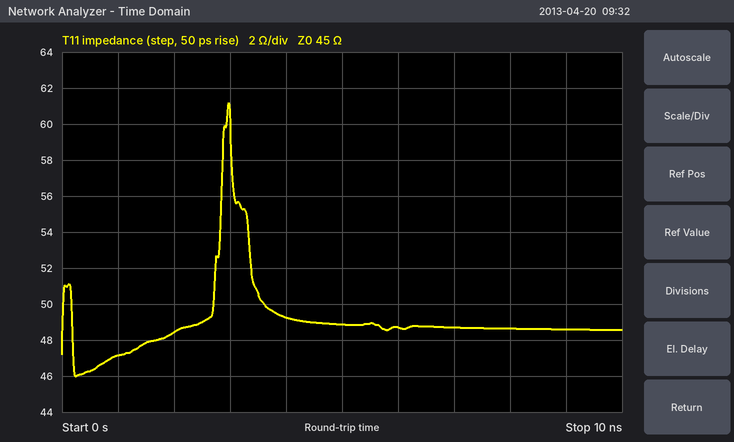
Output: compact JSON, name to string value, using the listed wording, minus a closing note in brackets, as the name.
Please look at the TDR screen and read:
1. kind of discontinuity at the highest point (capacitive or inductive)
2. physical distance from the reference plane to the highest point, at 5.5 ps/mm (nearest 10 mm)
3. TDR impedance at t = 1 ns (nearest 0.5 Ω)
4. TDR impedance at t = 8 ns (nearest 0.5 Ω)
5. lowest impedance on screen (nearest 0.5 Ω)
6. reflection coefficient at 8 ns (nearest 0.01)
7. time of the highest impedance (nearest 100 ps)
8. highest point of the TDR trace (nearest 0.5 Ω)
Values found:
{"kind of discontinuity at the highest point": "inductive", "physical distance from the reference plane to the highest point, at 5.5 ps/mm": "270 mm", "TDR impedance at t = 1 ns": "47.0 Ω", "TDR impedance at t = 8 ns": "48.5 Ω", "lowest impedance on screen": "46.0 Ω", "reflection coefficient at 8 ns": "+0.04", "time of the highest impedance": "3.0 ns", "highest point of the TDR trace": "61.0 Ω"}
